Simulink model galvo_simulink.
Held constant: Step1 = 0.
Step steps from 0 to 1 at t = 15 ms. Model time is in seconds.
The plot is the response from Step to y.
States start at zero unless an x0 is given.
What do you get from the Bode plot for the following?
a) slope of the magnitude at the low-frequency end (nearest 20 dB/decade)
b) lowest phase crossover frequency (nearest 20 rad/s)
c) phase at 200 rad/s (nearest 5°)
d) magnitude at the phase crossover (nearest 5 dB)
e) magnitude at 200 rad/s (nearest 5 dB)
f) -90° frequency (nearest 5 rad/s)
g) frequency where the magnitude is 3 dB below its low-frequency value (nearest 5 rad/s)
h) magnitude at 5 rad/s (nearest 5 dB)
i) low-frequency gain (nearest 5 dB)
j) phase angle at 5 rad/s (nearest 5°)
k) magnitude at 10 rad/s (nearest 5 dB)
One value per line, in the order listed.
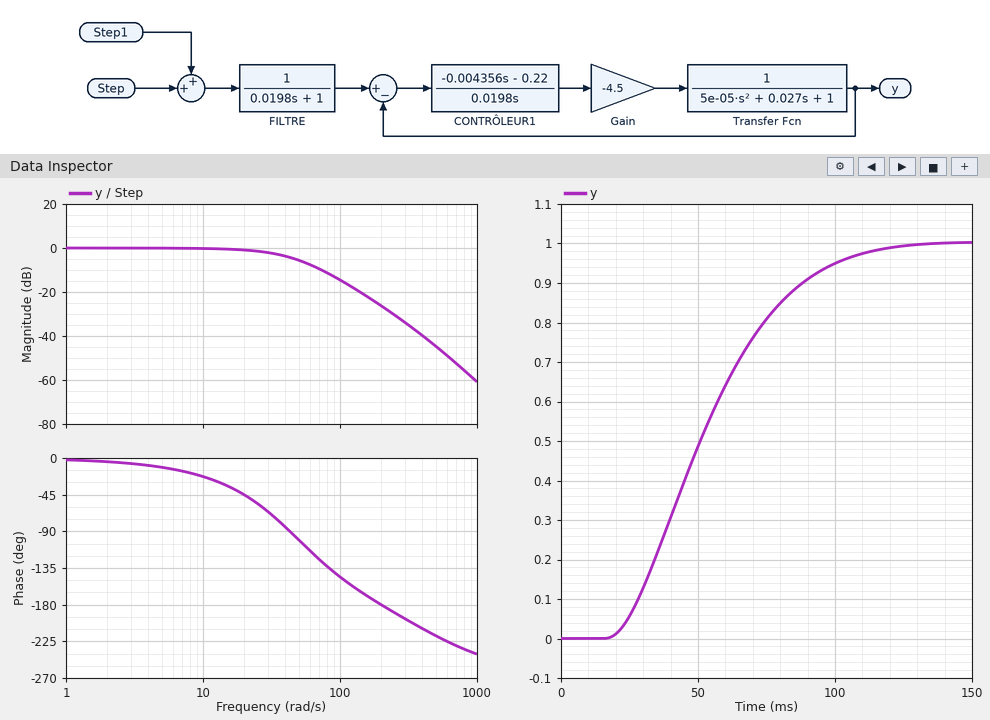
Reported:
0 dB/decade
200 rad/s
-180°
-25 dB
-25 dB
45 rad/s
35 rad/s
0 dB
0 dB
-10°
0 dB
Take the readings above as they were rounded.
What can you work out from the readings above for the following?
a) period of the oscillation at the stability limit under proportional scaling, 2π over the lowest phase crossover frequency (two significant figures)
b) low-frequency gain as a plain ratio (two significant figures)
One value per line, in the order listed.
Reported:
0.031 s
1.0
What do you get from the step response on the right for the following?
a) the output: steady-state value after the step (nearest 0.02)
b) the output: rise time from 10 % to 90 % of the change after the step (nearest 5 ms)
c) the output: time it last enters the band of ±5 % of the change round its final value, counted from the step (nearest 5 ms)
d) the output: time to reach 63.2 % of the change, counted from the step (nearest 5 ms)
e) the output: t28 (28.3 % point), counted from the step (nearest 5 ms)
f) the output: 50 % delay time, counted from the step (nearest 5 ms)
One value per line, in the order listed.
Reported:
1.00
60 ms
85 ms
45 ms
25 ms
35 ms
